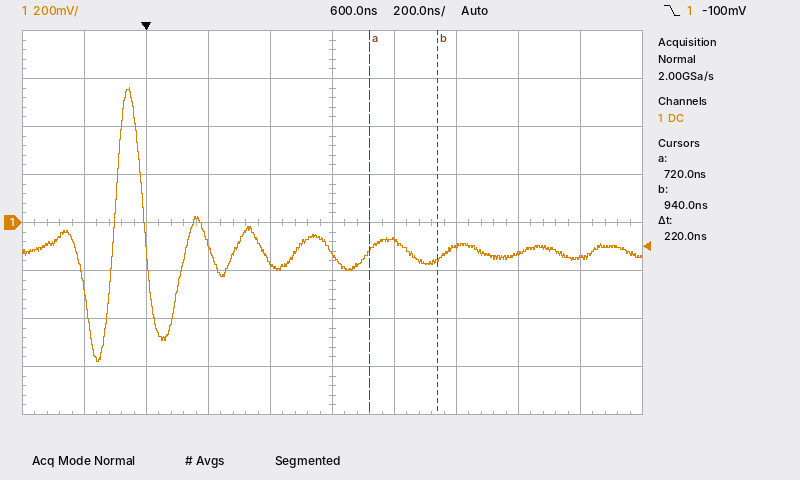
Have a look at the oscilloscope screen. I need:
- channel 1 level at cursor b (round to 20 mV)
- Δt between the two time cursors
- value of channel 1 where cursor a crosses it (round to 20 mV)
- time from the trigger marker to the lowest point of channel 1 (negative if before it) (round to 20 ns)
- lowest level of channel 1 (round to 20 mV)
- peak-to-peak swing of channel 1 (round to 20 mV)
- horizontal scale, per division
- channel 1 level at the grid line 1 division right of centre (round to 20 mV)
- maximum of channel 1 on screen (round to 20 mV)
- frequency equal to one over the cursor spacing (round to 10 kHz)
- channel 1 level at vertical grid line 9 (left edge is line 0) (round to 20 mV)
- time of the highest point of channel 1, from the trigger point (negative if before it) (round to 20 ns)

-160 mV
220 ns
-120 mV
-160 ns
-580 mV
1.14 V
200 ns
-80 mV
560 mV
4.55 MHz
-140 mV
-60 ns
